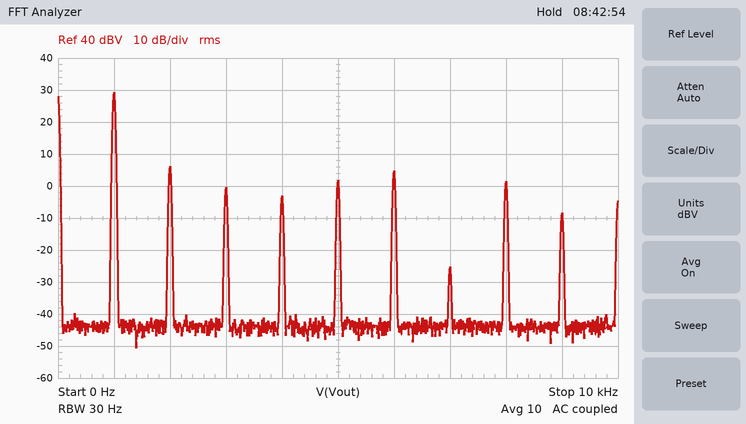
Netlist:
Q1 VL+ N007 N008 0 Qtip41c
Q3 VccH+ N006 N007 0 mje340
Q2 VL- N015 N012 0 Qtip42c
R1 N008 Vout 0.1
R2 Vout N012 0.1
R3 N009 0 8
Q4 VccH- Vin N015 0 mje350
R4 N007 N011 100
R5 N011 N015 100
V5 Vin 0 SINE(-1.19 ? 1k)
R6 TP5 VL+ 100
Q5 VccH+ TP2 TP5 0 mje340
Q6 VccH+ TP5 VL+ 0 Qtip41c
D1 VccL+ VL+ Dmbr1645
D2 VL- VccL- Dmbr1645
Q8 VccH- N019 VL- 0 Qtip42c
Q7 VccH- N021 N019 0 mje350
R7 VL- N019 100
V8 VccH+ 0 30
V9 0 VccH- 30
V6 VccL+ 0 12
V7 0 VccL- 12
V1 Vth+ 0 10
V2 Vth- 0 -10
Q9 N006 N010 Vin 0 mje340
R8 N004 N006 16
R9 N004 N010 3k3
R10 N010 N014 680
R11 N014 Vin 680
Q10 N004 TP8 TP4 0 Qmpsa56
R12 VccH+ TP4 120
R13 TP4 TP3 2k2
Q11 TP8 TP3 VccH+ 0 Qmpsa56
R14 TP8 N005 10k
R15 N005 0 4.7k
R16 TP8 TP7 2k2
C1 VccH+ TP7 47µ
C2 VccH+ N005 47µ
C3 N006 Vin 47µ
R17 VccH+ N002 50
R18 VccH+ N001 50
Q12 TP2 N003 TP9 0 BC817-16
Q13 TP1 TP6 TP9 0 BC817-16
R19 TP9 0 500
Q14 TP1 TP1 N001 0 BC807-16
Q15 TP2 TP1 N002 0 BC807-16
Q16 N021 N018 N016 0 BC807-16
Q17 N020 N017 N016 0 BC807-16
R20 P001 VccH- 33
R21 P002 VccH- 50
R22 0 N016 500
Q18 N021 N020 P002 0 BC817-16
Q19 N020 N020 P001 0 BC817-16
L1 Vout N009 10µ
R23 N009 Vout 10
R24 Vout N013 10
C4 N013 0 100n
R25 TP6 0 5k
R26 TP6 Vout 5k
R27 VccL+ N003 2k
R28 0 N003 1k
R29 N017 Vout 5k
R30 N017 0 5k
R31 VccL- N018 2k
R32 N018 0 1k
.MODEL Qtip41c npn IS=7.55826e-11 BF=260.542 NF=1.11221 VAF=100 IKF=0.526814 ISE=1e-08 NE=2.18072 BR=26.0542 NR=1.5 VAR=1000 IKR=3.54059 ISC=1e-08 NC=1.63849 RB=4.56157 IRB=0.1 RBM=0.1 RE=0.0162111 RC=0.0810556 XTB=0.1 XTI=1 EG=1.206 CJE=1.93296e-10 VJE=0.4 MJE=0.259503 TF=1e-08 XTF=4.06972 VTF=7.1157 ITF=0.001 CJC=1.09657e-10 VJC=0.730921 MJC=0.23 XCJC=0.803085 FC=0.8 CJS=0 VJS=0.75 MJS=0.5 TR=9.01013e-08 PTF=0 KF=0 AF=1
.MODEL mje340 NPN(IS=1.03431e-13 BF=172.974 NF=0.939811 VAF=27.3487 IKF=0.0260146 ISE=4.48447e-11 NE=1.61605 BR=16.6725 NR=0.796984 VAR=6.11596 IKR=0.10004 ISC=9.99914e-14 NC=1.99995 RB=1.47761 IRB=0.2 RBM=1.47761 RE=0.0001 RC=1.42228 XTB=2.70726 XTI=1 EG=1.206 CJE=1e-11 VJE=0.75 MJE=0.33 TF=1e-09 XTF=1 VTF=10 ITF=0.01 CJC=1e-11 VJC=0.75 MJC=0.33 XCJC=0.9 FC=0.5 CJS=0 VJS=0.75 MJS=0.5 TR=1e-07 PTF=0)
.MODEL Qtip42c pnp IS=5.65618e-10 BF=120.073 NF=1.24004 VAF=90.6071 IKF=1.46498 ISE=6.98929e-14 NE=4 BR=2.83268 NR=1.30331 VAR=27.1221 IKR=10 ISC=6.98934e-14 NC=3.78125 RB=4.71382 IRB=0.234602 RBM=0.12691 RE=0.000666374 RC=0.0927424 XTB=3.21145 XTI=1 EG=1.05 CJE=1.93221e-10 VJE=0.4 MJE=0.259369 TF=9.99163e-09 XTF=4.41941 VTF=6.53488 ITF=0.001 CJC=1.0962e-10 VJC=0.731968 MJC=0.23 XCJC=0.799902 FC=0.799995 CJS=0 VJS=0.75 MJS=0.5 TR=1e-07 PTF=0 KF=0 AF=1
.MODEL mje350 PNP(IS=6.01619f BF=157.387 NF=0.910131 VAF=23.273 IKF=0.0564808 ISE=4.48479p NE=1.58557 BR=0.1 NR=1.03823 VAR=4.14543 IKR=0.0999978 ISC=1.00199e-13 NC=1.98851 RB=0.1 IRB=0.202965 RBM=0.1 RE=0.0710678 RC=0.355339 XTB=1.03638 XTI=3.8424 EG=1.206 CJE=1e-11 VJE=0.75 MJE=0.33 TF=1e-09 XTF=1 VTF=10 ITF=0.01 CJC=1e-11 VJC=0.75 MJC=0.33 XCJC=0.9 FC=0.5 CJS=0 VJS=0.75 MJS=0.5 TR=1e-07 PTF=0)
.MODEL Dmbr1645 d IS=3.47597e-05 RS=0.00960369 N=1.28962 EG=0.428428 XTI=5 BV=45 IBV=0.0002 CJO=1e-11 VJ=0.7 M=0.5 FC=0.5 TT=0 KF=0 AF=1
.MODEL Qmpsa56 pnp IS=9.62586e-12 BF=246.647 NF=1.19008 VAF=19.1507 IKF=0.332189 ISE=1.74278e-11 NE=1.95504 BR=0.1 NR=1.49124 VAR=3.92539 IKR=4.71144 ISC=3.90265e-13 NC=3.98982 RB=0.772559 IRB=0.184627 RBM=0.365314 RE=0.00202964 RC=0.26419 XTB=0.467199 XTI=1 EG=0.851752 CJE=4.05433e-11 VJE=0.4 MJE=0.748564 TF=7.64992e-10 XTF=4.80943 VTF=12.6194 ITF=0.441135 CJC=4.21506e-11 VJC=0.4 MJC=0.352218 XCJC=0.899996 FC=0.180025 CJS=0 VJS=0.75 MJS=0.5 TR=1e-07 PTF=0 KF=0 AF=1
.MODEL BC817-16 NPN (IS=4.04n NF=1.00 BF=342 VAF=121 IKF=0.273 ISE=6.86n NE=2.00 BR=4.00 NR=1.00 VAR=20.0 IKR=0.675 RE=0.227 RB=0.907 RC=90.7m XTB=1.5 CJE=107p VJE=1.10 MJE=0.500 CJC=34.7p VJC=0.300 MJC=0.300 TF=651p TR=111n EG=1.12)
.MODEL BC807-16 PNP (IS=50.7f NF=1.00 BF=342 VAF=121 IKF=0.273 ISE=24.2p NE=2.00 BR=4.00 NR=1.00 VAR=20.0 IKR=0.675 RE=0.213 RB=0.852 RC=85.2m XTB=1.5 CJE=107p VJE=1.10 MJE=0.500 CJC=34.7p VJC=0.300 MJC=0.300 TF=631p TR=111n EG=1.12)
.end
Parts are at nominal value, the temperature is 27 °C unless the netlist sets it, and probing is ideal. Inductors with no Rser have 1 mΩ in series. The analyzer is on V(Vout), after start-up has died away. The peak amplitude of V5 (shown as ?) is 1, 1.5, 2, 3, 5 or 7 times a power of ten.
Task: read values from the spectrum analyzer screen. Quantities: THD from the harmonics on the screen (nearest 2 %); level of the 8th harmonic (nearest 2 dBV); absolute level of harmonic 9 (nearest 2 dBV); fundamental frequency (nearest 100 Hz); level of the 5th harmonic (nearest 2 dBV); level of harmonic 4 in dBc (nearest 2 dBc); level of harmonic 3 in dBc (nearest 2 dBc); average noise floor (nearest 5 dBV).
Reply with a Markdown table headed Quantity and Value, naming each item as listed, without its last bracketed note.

| Quantity | Value |
|---|---|
| THD from the harmonics on the screen | 12 % |
| level of the 8th harmonic | 2 dBV |
| absolute level of harmonic 9 | -8 dBV |
| fundamental frequency | 1.0 kHz |
| level of the 5th harmonic | 2 dBV |
| level of harmonic 4 in dBc | -32 dBc |
| level of harmonic 3 in dBc | -30 dBc |
| average noise floor | -45 dBV |
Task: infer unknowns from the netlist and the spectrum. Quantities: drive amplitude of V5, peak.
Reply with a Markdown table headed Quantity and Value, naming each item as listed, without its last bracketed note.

| Quantity | Value |
|---|---|
| drive amplitude of V5, peak | 70 V |
